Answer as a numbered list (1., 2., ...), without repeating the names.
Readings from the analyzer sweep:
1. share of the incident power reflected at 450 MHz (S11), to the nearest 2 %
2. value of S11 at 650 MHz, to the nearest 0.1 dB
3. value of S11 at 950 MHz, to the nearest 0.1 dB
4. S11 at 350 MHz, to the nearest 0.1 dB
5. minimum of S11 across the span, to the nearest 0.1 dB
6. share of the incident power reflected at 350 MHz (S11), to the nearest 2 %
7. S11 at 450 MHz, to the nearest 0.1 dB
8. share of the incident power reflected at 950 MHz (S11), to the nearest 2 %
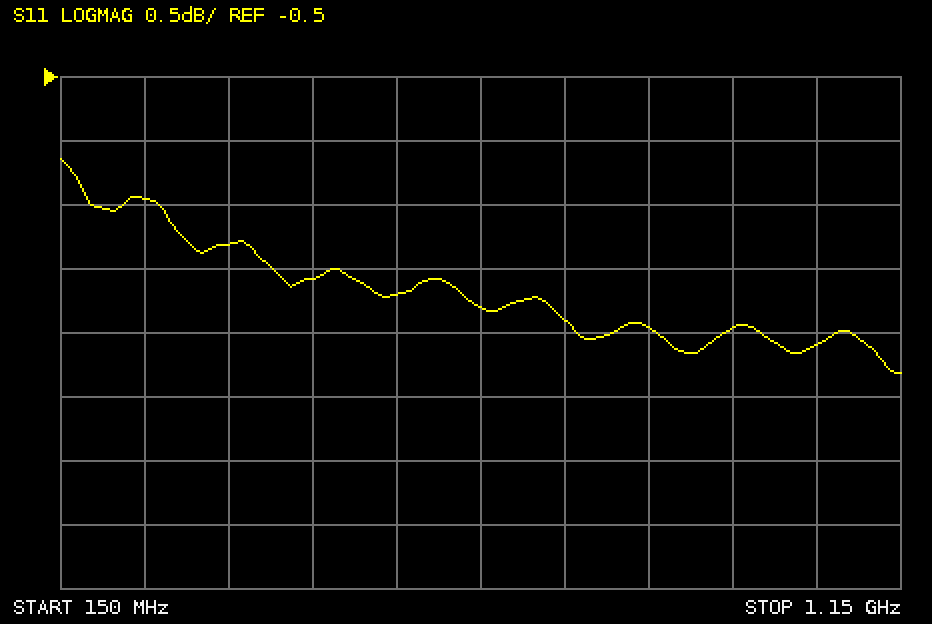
1. 62 %
2. -2.3 dB
3. -2.5 dB
4. -1.8 dB
5. -2.8 dB
6. 66 %
7. -2.1 dB
8. 56 %
